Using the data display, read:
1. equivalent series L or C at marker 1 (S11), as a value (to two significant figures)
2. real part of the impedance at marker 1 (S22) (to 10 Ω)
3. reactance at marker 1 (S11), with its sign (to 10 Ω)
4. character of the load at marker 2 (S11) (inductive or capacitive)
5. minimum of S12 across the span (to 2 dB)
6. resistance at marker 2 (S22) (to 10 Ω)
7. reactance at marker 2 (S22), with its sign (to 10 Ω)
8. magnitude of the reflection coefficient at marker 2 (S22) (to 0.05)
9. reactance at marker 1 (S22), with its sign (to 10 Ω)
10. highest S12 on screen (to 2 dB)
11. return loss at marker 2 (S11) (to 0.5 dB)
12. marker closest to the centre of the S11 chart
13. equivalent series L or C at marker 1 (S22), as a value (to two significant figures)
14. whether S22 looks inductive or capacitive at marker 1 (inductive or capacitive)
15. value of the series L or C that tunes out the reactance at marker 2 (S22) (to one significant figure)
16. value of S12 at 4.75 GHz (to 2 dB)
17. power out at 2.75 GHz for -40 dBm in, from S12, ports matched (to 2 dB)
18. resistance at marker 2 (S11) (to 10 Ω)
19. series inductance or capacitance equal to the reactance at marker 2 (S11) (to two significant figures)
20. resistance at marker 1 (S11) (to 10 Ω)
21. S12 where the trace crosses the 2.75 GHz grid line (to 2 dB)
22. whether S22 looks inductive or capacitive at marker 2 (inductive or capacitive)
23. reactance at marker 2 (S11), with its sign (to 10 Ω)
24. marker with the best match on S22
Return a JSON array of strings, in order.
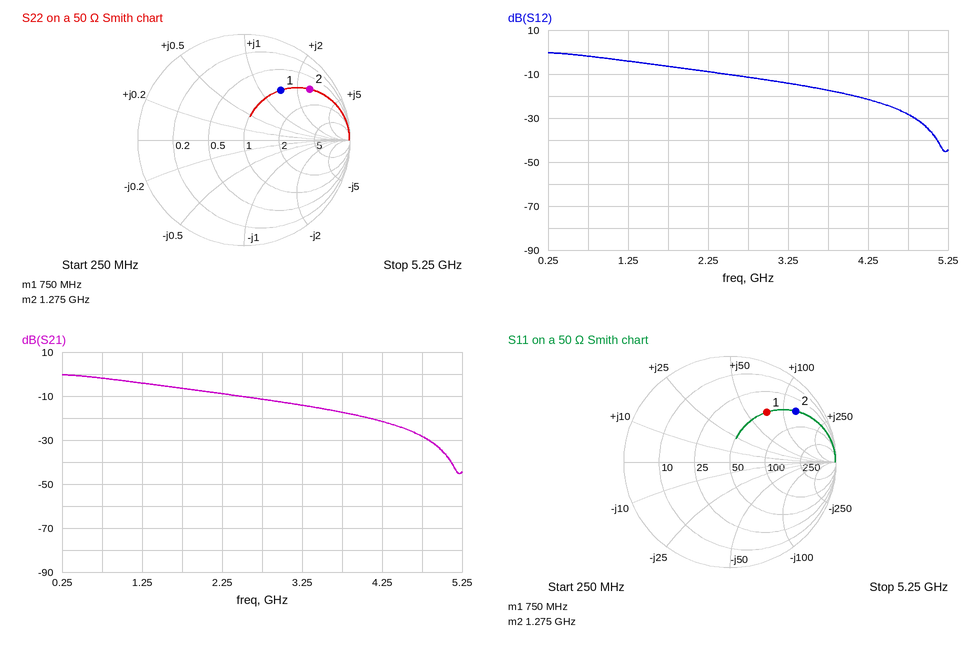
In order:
["15 nH", "50 Ω", "+70 Ω", "inductive", "-46 dB", "50 Ω", "+130 Ω", "0.80", "+70 Ω", "0 dB", "2.0 dB", "marker 1", "15 nH", "inductive", "1.0 pF", "-28 dB", "-52 dBm", "50 Ω", "16 nH", "50 Ω", "-12 dB", "inductive", "+130 Ω", "marker 1"]
